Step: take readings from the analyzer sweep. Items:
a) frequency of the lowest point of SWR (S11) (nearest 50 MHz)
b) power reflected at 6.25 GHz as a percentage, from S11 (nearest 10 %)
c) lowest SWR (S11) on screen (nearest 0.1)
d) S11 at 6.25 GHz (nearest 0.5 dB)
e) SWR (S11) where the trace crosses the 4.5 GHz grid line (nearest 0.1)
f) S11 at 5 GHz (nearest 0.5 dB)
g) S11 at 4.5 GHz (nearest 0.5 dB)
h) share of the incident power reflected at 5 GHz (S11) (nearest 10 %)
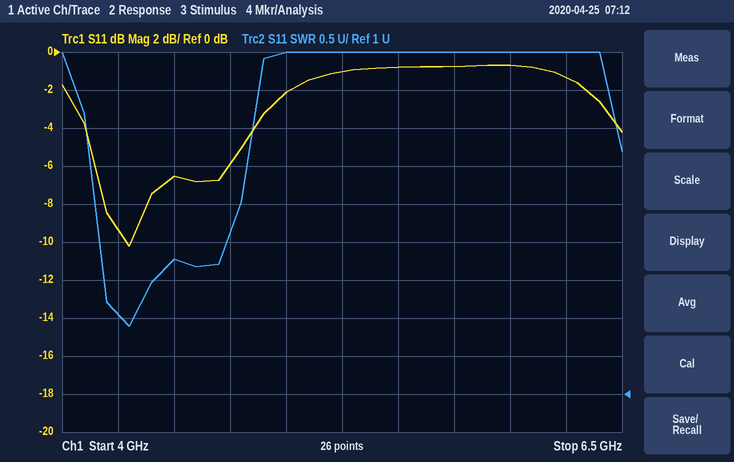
4.30 GHz
70 %
1.9
-1.5 dB
2.8
-2.0 dB
-6.5 dB
60 %
